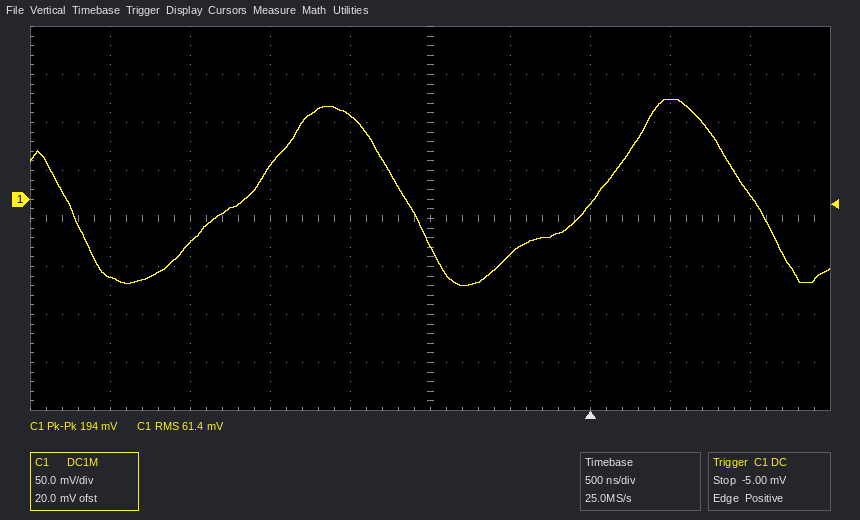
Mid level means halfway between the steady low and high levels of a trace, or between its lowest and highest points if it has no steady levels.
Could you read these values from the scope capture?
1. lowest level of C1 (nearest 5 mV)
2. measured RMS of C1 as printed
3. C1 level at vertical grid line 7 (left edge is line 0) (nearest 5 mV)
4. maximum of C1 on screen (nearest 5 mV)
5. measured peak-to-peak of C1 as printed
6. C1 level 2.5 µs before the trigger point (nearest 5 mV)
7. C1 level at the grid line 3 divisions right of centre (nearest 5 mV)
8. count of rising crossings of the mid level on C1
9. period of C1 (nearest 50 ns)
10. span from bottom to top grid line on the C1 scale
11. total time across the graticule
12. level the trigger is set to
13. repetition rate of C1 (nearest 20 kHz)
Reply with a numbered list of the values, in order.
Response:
1. -90 mV
2. 61.4 mV
3. -5 mV
4. 105 mV
5. 194 mV
6. -45 mV
7. 105 mV
8. 2
9. 2.15 µs
10. 400 mV
11. 5 µs
12. -5.00 mV
13. 460 kHz
